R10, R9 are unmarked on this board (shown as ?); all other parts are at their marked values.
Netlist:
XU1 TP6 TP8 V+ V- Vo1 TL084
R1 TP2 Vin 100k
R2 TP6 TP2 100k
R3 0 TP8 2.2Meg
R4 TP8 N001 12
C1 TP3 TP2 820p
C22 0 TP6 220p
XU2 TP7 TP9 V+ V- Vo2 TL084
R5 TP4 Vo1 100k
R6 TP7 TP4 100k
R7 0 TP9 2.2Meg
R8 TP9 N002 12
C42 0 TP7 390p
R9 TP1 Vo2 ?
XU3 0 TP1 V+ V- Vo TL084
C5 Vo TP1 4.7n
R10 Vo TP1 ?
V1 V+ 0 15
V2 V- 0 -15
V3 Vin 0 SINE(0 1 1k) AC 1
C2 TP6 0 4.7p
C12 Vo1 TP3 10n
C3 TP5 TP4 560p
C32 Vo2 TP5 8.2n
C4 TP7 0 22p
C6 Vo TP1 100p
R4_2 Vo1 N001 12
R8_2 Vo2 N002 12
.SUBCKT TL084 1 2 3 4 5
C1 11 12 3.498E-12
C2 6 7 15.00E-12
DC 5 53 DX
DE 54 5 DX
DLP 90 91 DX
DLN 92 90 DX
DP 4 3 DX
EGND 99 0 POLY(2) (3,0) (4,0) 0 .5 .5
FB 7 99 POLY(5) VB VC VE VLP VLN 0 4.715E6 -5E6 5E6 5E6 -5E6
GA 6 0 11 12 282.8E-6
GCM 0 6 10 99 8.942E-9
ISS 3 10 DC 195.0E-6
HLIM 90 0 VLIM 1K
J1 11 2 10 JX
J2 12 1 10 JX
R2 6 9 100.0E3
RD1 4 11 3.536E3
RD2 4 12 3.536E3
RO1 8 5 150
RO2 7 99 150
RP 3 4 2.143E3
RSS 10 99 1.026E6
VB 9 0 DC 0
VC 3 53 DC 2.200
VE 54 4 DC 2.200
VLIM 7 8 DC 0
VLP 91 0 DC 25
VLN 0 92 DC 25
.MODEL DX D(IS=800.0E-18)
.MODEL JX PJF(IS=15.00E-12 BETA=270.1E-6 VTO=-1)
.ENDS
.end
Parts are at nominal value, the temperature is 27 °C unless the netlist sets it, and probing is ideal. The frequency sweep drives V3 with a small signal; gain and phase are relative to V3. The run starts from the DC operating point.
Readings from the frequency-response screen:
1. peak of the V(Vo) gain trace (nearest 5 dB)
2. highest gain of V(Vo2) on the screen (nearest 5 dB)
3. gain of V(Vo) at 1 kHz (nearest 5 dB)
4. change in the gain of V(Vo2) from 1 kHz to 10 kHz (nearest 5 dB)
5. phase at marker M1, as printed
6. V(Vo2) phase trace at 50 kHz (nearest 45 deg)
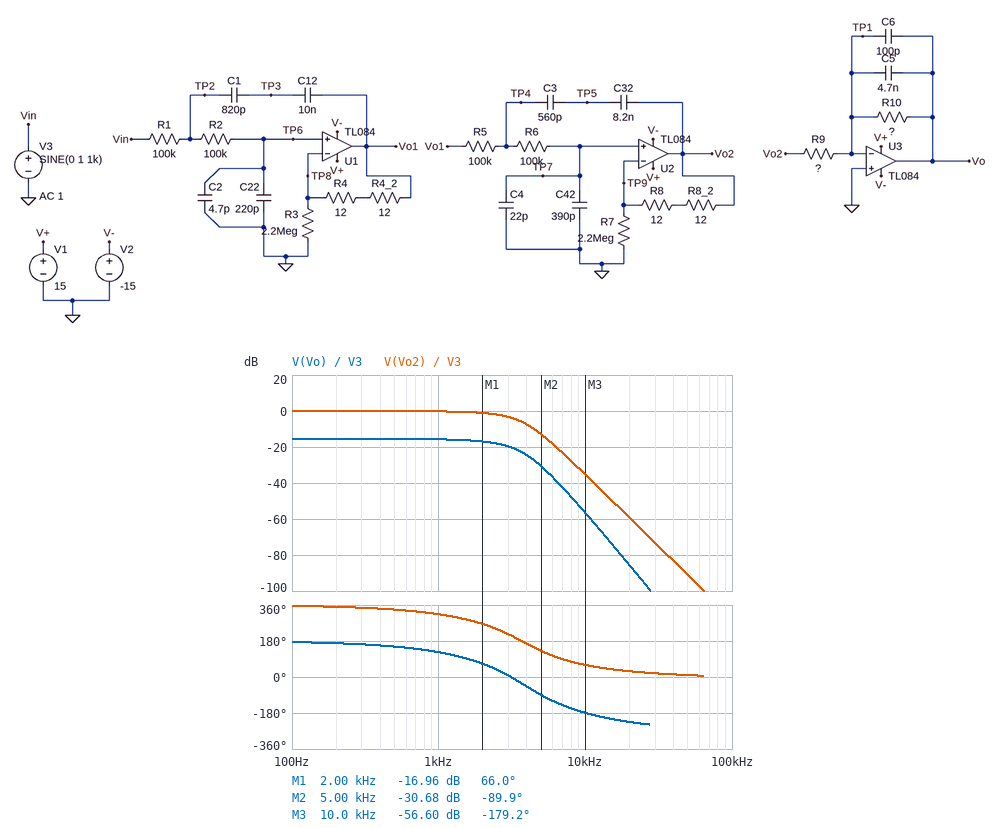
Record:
-15 dB
0 dB
-15 dB
-35 dB
66.0 deg
0 deg
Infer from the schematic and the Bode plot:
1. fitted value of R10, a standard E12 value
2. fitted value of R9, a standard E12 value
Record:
5.6 kΩ
33 kΩ
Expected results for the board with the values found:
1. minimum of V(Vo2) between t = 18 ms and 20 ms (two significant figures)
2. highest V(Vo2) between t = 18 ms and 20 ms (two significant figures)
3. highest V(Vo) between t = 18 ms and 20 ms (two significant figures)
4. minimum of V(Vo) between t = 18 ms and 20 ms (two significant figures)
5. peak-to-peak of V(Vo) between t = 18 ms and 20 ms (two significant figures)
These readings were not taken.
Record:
-980 mV
980 mV
160 mV
-160 mV
330 mV
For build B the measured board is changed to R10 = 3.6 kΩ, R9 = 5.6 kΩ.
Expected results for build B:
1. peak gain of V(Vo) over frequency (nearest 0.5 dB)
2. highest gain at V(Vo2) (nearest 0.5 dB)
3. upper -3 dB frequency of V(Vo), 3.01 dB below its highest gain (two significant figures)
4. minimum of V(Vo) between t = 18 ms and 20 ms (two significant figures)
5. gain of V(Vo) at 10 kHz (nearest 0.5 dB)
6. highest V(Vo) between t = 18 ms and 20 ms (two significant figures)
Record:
-4.0 dB
0 dB
2.8 kHz
-620 mV
-42.5 dB
620 mV
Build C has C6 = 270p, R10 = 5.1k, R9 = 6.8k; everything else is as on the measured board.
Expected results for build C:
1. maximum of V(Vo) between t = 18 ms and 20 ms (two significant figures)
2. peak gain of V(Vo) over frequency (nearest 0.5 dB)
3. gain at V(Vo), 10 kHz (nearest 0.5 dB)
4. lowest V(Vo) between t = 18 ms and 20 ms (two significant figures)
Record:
720 mV
-2.5 dB
-43.5 dB
-720 mV
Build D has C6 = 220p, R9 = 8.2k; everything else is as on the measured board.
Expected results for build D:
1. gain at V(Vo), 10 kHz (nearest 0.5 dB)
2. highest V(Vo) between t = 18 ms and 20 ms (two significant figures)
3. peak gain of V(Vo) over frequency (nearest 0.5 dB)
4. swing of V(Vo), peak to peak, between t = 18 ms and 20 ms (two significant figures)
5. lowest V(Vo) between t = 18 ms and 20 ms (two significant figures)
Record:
-44.5 dB
660 mV
-3.5 dB
1.3 V
-660 mV
